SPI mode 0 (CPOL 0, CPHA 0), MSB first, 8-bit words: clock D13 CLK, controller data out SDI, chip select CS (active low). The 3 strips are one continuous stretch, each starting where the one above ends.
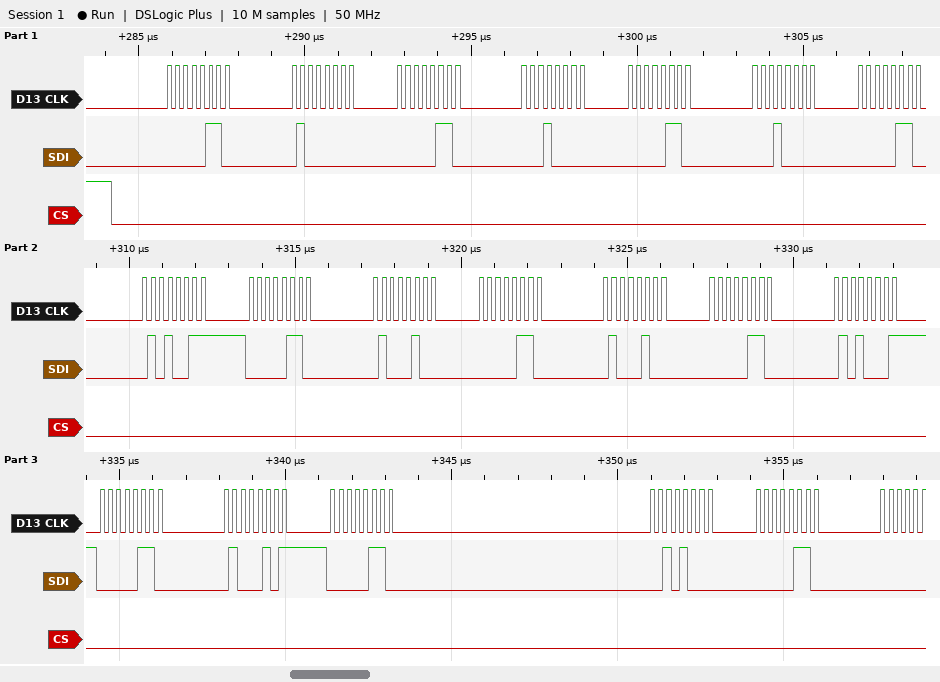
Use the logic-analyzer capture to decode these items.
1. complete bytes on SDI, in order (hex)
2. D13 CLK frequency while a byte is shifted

06 40 06 10 06 10 06 53 06 44 06 44 06 51 06 45 06 28 06
4 MHz
